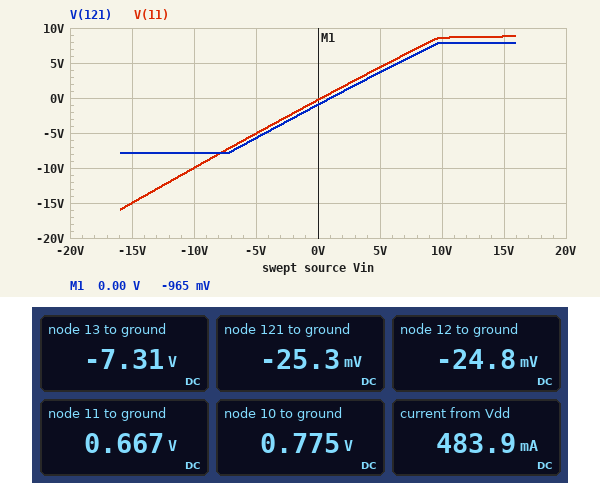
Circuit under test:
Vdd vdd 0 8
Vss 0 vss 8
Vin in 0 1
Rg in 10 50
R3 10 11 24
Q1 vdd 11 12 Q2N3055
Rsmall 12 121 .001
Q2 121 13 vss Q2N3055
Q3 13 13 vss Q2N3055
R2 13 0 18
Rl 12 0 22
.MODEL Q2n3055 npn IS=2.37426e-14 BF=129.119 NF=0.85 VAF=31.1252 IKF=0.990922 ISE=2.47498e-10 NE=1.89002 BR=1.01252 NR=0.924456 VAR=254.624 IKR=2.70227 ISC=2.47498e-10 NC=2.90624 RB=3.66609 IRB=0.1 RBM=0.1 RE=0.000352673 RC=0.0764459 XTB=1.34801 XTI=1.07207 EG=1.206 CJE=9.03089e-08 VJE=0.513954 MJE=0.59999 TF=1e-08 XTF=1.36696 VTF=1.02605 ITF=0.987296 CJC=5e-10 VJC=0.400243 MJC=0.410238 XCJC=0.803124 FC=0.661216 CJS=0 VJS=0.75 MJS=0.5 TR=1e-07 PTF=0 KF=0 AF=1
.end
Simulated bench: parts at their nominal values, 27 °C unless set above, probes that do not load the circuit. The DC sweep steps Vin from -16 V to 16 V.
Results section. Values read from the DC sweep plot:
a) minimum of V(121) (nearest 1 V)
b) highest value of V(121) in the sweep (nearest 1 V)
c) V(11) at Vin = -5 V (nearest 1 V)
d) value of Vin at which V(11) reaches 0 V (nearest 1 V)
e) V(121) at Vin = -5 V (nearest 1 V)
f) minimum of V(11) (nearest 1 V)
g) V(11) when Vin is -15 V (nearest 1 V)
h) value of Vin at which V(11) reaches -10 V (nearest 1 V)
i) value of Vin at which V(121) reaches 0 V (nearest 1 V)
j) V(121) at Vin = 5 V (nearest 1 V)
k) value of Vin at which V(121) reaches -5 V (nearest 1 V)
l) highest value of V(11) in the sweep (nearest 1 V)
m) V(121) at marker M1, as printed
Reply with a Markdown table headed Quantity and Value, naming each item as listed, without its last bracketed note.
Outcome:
| Quantity | Value |
|---|---|
| minimum of V(121) | -8 V |
| highest value of V(121) in the sweep | 8 V |
| V(11) at Vin = -5 V | -5 V |
| value of Vin at which V(11) reaches 0 V | 0 V |
| V(121) at Vin = -5 V | -6 V |
| minimum of V(11) | -16 V |
| V(11) when Vin is -15 V | -15 V |
| value of Vin at which V(11) reaches -10 V | -10 V |
| value of Vin at which V(121) reaches 0 V | 1 V |
| V(121) at Vin = 5 V | 4 V |
| value of Vin at which V(121) reaches -5 V | -4 V |
| highest value of V(11) in the sweep | 9 V |
| V(121) at marker M1, as printed | -965 mV |
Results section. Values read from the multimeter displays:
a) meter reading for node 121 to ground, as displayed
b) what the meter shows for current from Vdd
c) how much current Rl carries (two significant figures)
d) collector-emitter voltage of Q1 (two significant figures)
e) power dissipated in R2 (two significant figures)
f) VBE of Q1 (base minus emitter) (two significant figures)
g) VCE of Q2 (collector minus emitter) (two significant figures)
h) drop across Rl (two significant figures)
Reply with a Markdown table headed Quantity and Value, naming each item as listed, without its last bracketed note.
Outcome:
| Quantity | Value |
|---|---|
| meter reading for node 121 to ground, as displayed | -25.3 mV |
| what the meter shows for current from Vdd | 483.9 mA |
| how much current Rl carries | 1.1 mA |
| collector-emitter voltage of Q1 | 8.0 V |
| power dissipated in R2 | 3.0 W |
| VBE of Q1 (base minus emitter) | 690 mV |
| VCE of Q2 (collector minus emitter) | 8.0 V |
| drop across Rl | 25 mV |
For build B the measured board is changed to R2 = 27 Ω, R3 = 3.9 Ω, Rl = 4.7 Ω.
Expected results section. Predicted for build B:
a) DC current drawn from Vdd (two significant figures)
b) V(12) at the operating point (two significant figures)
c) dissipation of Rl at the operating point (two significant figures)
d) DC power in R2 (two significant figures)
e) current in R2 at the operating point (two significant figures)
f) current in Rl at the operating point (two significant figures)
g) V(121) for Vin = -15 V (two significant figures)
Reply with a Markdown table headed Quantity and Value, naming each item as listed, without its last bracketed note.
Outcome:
| Quantity | Value |
|---|---|
| DC current drawn from Vdd | 360 mA |
| V(12) at the operating point | 150 mV |
| dissipation of Rl at the operating point | 4.9 mW |
| DC power in R2 | 2.0 W |
| current in R2 at the operating point | 270 mA |
| current in Rl at the operating point | 32 mA |
| V(121) for Vin = -15 V | -1.5 V |
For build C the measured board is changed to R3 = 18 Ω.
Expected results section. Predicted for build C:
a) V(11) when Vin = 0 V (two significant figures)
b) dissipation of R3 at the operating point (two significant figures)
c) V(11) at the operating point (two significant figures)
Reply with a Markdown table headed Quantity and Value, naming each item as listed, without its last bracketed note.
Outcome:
| Quantity | Value |
|---|---|
| V(11) when Vin = 0 V | -260 mV |
| dissipation of R3 at the operating point | 370 µW |
| V(11) at the operating point | 690 mV |
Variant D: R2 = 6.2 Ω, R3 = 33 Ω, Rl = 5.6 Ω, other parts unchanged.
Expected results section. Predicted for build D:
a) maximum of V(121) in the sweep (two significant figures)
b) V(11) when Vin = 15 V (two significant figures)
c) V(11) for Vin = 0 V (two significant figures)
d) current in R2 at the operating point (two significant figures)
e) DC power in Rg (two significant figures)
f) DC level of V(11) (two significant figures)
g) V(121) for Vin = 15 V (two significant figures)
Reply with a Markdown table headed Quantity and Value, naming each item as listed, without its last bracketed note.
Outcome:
| Quantity | Value |
|---|---|
| maximum of V(121) in the sweep | 7.5 V |
| V(11) when Vin = 15 V | 7.9 V |
| V(11) for Vin = 0 V | -950 mV |
| current in R2 at the operating point | 1.2 A |
| DC power in Rg | 10 mW |
| DC level of V(11) | -200 mV |
| V(121) for Vin = 15 V | 7.0 V |
